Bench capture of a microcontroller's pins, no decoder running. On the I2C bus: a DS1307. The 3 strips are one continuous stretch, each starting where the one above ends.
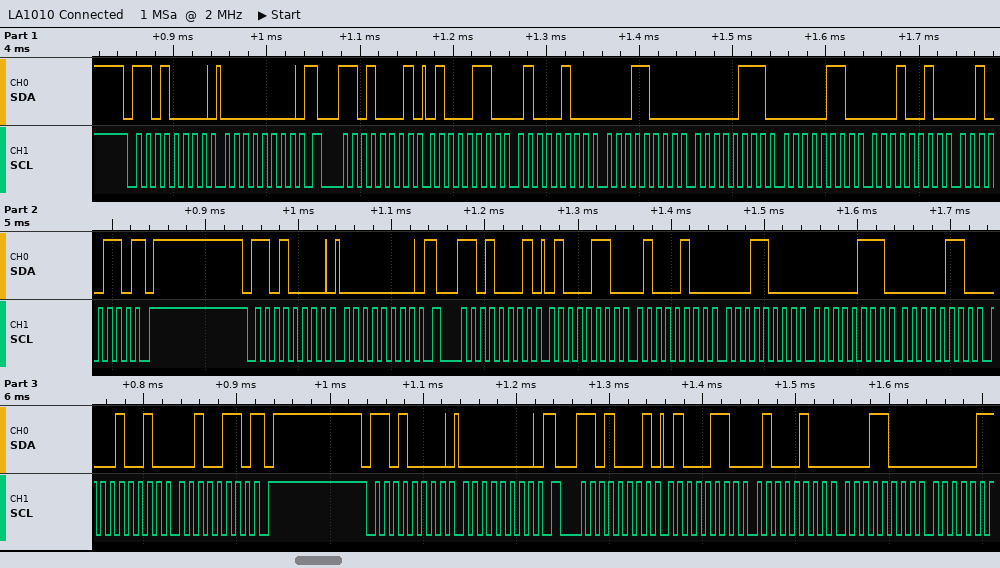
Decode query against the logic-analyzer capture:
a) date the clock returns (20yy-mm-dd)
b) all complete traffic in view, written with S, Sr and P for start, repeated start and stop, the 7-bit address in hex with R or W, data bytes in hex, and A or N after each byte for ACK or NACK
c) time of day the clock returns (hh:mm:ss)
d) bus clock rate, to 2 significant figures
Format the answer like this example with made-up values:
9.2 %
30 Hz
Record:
2026-12-06
S 68W A 00 A Sr 68R A 46 A 44 A 18 A 07 A 06 A 12 A 26 N P S 68W A 00 A Sr 68R A 46 A 44 A 18 A 07 A 06 A 12 A 26 N P S 68W A 00 A Sr 68R A 46 A 44 A 18 A
18:44:46
100 kHz
